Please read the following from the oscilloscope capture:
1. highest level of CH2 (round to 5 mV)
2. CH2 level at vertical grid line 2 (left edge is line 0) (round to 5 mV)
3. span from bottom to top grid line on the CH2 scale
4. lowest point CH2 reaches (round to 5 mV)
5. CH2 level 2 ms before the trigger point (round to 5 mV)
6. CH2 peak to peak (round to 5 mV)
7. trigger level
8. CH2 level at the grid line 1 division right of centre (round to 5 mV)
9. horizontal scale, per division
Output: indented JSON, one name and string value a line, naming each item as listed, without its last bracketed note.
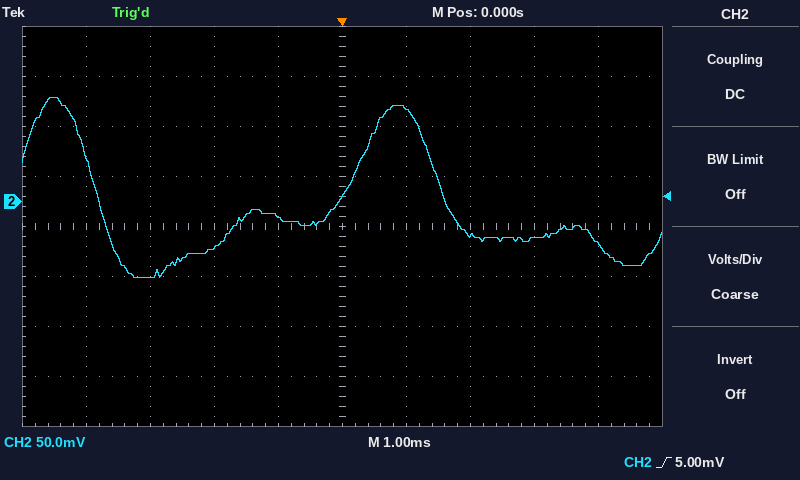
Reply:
{
  "highest level of CH2": "105 mV",
  "CH2 level at vertical grid line 2 (left edge is line 0)": "-75 mV",
  "span from bottom to top grid line on the CH2 scale": "400 mV",
  "lowest point CH2 reaches": "-75 mV",
  "CH2 level 2 ms before the trigger point": "-45 mV",
  "CH2 peak to peak": "180 mV",
  "trigger level": "5.00 mV",
  "CH2 level at the grid line 1 division right of centre": "95 mV",
  "horizontal scale, per division": "1 ms"
}
